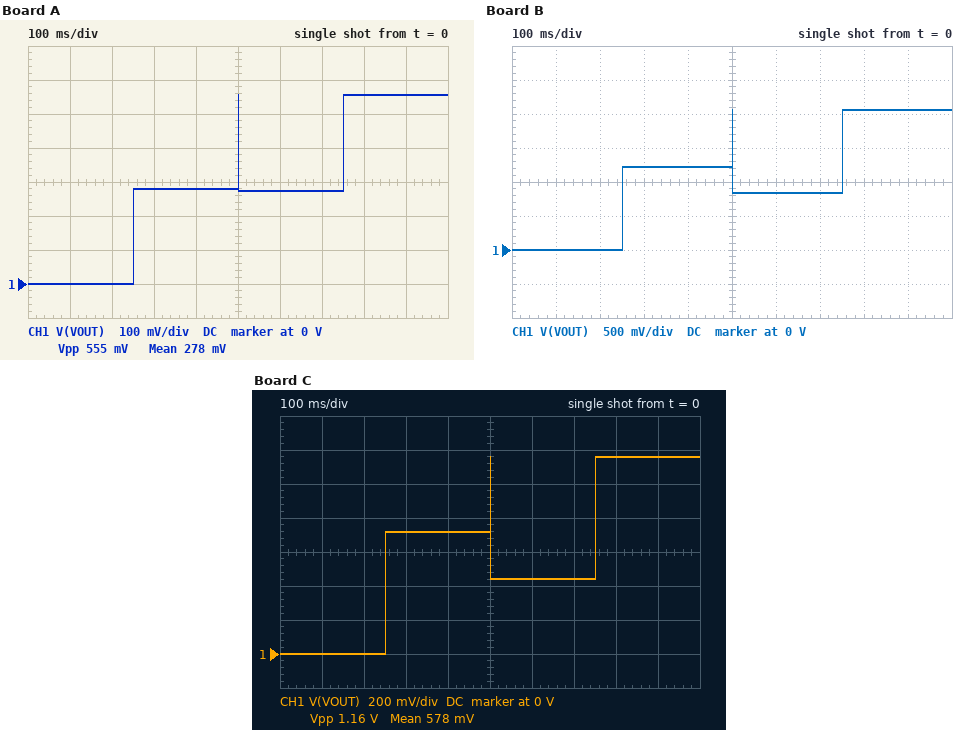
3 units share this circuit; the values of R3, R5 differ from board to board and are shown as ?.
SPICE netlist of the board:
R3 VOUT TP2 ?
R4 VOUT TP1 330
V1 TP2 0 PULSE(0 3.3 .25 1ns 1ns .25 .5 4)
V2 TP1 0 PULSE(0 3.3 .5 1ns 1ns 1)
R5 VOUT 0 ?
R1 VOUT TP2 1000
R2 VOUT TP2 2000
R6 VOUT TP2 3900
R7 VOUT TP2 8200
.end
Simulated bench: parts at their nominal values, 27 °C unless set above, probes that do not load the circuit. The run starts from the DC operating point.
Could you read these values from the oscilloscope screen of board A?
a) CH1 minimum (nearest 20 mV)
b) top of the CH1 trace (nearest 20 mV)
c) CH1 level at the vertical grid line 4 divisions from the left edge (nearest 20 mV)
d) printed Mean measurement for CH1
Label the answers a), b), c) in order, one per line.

a) 0 V
b) 560 mV
c) 280 mV
d) 278 mV
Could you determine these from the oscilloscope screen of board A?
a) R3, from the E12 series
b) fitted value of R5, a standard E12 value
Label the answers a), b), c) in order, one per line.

a) 820 Ω
b) 33 Ω
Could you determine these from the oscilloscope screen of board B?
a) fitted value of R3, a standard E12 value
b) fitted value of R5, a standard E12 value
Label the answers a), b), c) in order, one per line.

a) 390 Ω
b) 220 Ω
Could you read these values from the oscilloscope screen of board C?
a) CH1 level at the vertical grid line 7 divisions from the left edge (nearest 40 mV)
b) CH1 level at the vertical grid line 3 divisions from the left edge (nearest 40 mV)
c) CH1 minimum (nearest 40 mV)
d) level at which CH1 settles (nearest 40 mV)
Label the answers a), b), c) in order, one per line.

a) 440 mV
b) 720 mV
c) 0 V
d) 1.16 V
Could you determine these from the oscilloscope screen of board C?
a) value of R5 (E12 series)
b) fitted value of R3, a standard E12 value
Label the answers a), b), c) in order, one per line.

a) 68 Ω
b) 330 Ω
